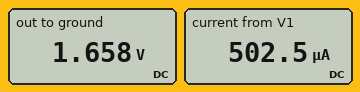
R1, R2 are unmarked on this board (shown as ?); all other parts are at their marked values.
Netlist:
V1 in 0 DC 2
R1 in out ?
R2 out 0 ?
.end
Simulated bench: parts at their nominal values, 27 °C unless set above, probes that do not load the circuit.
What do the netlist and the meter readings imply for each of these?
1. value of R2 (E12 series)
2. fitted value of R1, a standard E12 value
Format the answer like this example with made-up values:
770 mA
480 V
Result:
3.3 kΩ
680 Ω
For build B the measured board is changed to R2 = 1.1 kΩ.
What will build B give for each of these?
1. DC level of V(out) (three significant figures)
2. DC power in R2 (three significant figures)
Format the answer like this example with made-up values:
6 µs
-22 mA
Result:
1.24 V
1.39 mW
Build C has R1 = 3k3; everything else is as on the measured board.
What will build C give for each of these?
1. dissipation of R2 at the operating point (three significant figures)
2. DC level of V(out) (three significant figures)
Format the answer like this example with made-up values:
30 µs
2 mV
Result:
303 µW
1.00 V
